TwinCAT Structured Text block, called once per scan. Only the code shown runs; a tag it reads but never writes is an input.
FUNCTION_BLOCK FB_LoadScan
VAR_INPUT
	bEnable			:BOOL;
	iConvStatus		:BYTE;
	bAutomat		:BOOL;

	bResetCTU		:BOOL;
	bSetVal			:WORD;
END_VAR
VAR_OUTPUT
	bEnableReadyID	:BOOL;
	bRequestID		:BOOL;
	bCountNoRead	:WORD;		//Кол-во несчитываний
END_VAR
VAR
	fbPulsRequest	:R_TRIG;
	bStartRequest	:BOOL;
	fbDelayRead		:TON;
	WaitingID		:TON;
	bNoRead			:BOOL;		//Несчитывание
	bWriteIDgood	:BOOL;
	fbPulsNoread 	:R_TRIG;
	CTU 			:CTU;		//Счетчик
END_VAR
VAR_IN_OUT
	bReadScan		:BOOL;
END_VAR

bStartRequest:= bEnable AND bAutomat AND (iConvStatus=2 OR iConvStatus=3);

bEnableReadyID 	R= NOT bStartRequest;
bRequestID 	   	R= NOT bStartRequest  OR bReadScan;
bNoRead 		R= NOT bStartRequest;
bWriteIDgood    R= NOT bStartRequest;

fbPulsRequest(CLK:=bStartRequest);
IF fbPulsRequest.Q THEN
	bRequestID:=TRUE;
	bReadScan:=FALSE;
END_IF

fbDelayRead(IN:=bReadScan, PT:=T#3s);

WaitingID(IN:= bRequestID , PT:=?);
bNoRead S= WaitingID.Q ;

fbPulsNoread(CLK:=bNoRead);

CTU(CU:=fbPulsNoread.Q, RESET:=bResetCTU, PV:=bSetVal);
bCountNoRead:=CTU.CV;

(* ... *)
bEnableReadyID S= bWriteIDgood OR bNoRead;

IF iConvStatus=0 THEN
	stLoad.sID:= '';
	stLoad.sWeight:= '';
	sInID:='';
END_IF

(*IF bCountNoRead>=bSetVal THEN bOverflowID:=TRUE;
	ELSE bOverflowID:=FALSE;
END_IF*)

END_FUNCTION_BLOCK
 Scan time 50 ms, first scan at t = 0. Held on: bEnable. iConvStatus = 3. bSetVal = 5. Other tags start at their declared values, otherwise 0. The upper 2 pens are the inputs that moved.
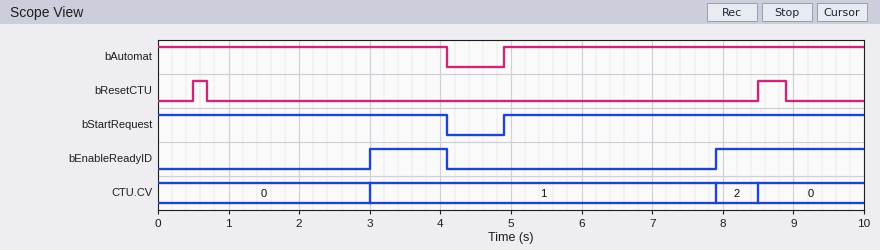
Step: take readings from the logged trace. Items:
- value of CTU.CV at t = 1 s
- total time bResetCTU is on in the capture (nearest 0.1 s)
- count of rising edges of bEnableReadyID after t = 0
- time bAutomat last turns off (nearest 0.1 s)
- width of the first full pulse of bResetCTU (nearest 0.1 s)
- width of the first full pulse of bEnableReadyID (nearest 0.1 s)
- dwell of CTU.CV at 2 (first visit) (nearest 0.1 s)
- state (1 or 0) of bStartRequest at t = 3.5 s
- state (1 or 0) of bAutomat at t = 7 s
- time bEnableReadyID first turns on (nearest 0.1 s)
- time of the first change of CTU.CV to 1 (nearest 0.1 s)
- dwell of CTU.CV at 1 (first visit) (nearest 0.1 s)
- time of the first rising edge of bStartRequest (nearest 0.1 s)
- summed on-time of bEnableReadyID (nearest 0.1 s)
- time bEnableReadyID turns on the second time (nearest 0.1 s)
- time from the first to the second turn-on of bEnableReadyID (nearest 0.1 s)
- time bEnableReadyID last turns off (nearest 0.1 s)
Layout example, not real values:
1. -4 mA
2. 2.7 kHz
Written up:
1. 0
2. 0.6 s
3. 2
4. 4.1 s
5. 0.2 s
6. 1.1 s
7. 0.6 s
8. 1
9. 1
10. 3.0 s
11. 3.0 s
12. 4.9 s
13. 4.9 s
14. 3.2 s
15. 7.9 s
16. 4.9 s
17. 4.1 s
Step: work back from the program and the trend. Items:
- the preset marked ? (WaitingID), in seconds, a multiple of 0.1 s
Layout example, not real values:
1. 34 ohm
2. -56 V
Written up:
1. 3.0 s
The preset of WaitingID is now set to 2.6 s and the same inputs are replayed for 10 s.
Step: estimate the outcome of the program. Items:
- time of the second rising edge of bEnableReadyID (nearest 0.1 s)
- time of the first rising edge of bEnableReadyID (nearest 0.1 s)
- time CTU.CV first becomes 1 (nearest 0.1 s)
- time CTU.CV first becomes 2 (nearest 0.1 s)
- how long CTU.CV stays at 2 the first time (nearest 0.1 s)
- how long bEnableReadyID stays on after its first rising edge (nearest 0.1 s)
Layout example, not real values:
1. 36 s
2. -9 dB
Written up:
1. 7.5 s
2. 2.6 s
3. 2.6 s
4. 7.5 s
5. 1.0 s
6. 1.5 s
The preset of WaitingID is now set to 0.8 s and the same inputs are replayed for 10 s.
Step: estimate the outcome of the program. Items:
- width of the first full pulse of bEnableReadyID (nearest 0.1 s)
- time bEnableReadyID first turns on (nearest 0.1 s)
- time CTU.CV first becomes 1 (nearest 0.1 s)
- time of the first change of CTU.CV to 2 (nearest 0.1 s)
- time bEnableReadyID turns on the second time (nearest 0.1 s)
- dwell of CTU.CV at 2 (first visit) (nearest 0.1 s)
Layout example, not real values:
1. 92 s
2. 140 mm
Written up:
1. 3.3 s
2. 0.8 s
3. 0.8 s
4. 5.7 s
5. 5.7 s
6. 2.8 s
